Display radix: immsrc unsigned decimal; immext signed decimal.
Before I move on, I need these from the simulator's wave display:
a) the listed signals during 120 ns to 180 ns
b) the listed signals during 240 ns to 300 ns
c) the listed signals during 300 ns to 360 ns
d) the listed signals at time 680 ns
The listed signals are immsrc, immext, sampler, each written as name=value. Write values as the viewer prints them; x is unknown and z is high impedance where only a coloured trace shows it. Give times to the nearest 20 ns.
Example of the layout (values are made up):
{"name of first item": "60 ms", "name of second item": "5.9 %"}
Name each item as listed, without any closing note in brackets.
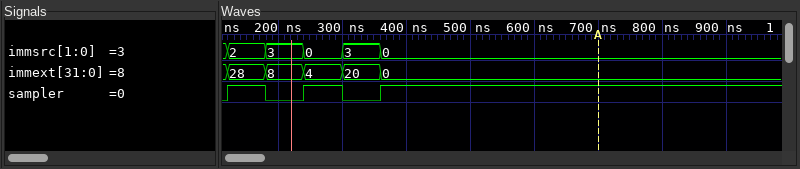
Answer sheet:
{"the listed signals during 120 ns to 180 ns": "immsrc=2, immext=28, sampler=1", "the listed signals during 240 ns to 300 ns": "immsrc=0, immext=4, sampler=1", "the listed signals during 300 ns to 360 ns": "immsrc=3, immext=20, sampler=0", "the listed signals at time 680 ns": "immsrc=0, immext=0, sampler=1"}
